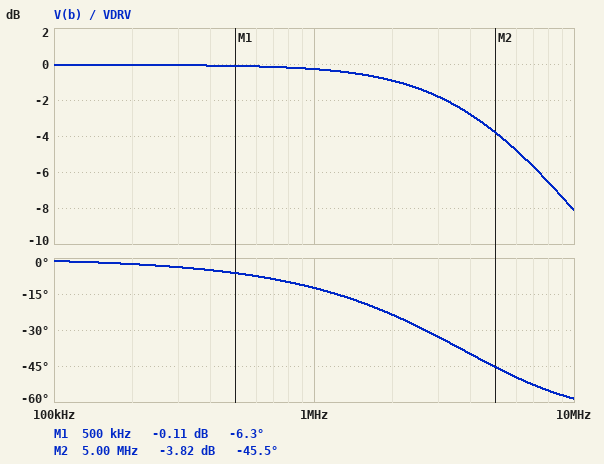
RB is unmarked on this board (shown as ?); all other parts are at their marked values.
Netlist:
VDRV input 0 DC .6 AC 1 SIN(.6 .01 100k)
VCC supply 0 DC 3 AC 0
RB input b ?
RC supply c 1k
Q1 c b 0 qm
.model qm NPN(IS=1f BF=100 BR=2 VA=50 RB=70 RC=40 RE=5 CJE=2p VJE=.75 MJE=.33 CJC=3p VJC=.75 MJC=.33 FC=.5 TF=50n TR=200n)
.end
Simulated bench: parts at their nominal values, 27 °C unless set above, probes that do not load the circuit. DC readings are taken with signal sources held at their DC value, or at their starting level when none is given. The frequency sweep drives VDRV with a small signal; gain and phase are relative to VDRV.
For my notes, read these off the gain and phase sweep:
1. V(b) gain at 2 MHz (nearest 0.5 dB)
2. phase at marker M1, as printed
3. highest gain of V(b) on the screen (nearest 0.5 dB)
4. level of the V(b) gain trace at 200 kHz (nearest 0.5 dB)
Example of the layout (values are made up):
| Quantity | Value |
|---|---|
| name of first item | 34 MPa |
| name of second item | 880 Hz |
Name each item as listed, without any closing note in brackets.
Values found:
| Quantity | Value |
|---|---|
| V(b) gain at 2 MHz | -1.0 dB |
| phase at marker M1, as printed | -6.3 deg |
| highest gain of V(b) on the screen | 0 dB |
| level of the V(b) gain trace at 200 kHz | 0 dB |
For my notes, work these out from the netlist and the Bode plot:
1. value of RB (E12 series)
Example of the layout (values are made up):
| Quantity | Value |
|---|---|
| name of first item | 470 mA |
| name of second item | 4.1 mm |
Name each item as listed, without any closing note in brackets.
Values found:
| Quantity | Value |
|---|---|
| value of RB | 1.2 kΩ |
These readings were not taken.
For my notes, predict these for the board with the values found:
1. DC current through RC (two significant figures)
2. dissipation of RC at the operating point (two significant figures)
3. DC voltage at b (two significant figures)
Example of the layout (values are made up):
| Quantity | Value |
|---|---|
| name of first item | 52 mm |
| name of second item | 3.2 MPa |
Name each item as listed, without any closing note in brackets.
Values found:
| Quantity | Value |
|---|---|
| DC current through RC | 12 µA |
| dissipation of RC at the operating point | 150 nW |
| DC voltage at b | 600 mV |
